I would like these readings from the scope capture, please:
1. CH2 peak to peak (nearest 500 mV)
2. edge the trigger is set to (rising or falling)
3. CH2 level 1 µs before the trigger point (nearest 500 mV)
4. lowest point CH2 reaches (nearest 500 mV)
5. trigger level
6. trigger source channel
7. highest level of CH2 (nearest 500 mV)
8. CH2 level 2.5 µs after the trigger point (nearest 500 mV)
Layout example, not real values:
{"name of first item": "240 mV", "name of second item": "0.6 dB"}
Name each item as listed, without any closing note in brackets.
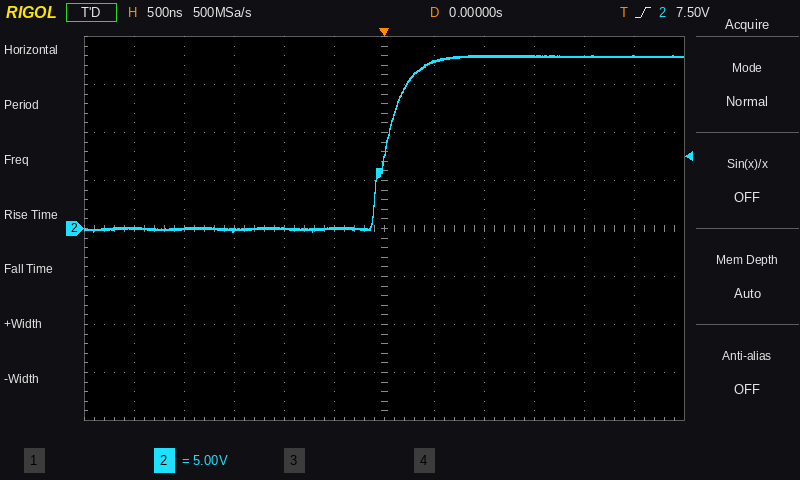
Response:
{"CH2 peak to peak": "18.5 V", "edge the trigger is set to": "rising", "CH2 level 1 µs before the trigger point": "0.0 V", "lowest point CH2 reaches": "-500 mV", "trigger level": "7.50 V", "trigger source channel": "CH2", "highest level of CH2": "18.0 V", "CH2 level 2.5 µs after the trigger point": "18.0 V"}
